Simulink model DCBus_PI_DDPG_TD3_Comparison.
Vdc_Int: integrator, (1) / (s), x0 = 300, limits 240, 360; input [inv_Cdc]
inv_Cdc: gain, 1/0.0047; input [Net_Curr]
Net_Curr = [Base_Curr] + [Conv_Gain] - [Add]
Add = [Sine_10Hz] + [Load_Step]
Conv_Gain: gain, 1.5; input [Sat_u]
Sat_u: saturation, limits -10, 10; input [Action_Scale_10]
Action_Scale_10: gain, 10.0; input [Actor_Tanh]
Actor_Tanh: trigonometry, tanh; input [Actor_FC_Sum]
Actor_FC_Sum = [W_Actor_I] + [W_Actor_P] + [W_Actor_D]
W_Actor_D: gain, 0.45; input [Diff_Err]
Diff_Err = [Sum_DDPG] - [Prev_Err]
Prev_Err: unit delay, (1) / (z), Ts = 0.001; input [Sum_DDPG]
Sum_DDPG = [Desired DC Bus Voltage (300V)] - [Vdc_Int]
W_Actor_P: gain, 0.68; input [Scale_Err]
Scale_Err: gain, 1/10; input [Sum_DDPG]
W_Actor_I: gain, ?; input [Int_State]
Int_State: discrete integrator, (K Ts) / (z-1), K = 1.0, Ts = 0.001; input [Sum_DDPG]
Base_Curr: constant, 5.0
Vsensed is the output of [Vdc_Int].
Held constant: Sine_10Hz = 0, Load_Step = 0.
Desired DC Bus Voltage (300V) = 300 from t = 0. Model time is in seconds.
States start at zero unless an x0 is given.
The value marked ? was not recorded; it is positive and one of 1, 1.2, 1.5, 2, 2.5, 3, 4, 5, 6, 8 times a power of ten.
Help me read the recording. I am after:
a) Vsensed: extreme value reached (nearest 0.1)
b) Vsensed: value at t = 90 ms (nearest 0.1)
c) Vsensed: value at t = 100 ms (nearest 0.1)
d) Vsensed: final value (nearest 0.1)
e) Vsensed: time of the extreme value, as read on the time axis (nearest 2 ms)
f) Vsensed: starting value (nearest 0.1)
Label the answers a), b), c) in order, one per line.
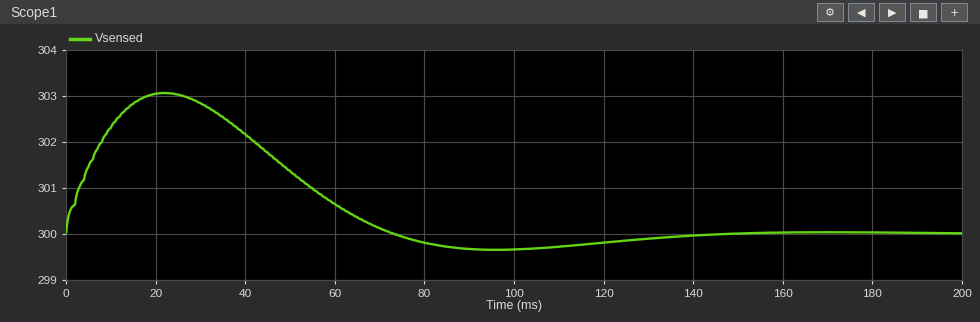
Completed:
a) 303.1
b) 299.7
c) 299.7
d) 300.0
e) 22 ms
f) 300.0
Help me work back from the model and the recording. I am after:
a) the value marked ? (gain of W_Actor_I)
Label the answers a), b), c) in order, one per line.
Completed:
a) 3
